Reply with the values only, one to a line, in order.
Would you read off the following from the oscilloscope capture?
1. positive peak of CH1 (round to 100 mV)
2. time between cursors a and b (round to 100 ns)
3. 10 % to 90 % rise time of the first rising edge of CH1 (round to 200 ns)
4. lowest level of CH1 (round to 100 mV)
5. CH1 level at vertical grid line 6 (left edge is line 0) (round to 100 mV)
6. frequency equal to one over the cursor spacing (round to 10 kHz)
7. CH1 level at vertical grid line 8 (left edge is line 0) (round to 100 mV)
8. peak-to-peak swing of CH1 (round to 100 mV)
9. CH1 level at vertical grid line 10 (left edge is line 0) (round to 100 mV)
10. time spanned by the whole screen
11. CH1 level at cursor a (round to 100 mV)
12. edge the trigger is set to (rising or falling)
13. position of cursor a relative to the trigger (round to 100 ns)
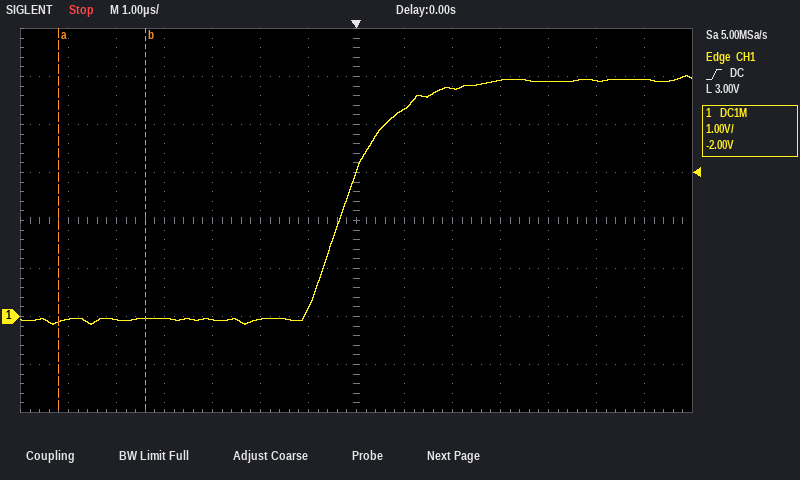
5.0 V
1.8 µs
2.0 µs
-200 mV
200 mV
560 kHz
4.3 V
5.2 V
4.9 V
14 µs
-100 mV
rising
-6.2 µs
